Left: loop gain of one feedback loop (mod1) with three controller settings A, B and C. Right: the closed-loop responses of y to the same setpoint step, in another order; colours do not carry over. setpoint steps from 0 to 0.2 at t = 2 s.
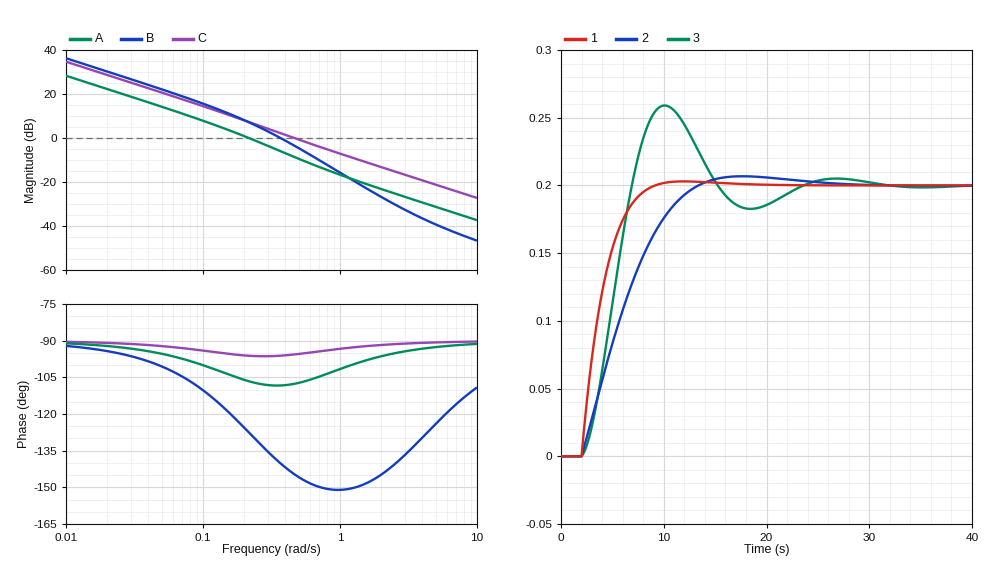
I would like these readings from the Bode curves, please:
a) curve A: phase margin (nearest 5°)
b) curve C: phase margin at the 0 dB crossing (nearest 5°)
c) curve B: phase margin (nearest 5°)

75°
85°
40°
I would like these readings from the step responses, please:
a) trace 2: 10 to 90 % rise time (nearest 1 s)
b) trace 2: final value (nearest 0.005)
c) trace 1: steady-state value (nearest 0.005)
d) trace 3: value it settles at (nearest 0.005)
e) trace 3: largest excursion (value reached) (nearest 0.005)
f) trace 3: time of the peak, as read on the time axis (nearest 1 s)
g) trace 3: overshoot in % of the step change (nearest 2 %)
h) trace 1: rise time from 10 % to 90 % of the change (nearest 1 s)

8 s
0.200
0.200
0.200
0.260
10 s
30 %
4 s
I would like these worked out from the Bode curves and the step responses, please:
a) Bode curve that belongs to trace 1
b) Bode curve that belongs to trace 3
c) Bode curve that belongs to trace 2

C
B
A
